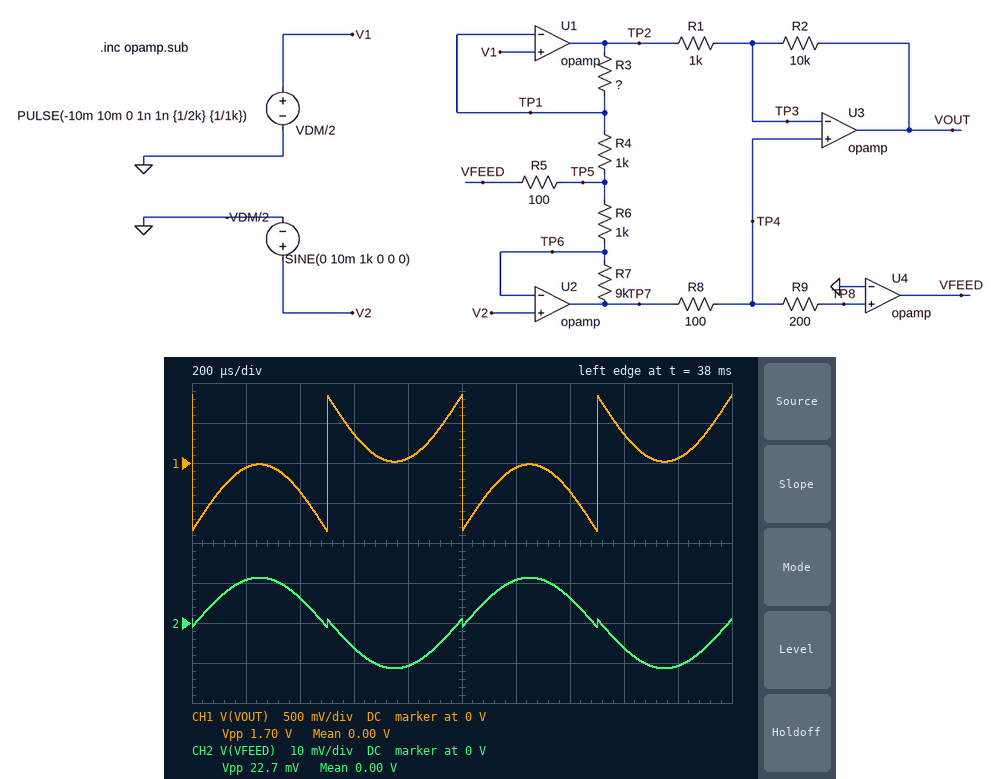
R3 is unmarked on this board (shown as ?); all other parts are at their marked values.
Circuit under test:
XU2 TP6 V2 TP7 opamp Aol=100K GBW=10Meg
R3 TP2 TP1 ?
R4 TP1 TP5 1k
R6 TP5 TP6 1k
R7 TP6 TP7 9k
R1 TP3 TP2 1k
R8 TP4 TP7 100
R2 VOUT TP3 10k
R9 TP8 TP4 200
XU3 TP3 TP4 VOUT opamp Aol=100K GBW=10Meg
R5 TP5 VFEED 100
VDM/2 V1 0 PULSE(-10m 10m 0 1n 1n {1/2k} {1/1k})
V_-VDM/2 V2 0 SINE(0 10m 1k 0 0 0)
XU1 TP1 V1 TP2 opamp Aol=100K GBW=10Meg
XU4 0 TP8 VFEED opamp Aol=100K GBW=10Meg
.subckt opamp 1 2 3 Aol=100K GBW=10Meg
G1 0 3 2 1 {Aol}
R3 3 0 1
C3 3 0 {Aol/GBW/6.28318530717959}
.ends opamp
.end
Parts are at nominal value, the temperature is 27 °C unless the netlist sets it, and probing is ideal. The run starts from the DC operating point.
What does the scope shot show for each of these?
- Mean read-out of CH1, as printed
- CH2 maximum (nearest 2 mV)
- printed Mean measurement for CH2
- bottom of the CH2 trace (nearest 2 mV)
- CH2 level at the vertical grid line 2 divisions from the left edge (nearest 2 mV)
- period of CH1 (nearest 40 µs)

0.00 V
12 mV
0.00 V
-12 mV
6 mV
1.00 ms
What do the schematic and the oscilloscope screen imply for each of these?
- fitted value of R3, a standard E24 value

7.5 kΩ
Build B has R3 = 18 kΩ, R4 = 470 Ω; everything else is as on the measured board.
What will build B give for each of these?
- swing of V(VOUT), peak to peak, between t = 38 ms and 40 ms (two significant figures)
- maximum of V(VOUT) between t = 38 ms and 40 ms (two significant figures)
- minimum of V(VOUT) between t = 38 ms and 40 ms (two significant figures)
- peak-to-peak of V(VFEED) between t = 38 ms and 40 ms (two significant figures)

7.8 V
3.9 V
-3.9 V
23 mV
